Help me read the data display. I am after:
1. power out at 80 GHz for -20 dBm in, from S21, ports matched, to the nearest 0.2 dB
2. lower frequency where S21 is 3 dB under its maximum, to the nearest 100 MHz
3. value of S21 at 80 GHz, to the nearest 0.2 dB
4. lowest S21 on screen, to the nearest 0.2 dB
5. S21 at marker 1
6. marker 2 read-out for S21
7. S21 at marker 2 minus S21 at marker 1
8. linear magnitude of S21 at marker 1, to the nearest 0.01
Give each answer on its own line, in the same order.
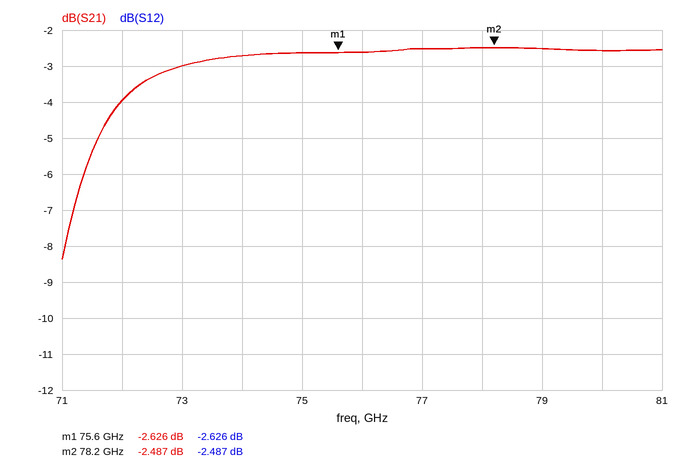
-22.6 dBm
71.5 GHz
-2.6 dB
-8.4 dB
-2.626 dB
-2.487 dB
0.139 dB
0.74
